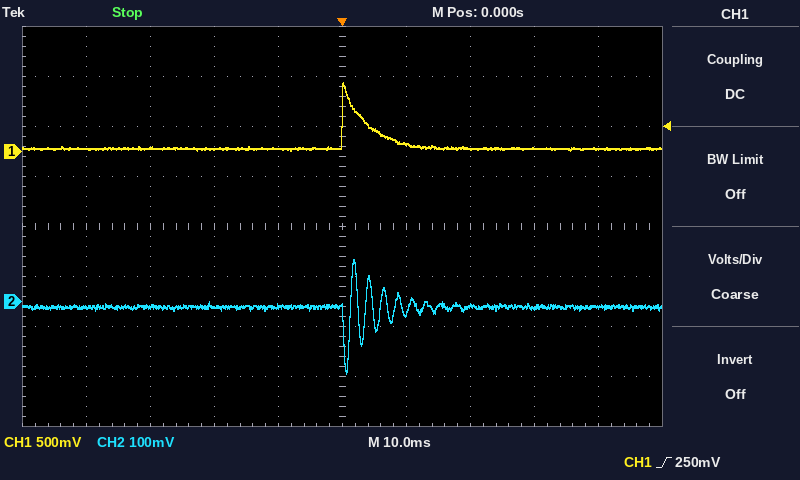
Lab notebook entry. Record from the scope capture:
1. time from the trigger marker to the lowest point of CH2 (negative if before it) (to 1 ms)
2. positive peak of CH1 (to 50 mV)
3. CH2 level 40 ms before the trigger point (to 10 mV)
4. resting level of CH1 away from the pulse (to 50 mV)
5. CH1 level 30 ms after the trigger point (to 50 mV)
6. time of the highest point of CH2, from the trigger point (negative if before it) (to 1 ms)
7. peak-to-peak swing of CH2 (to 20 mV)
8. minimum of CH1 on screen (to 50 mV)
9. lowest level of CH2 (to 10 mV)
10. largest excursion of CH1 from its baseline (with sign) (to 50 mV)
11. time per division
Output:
+1 ms
700 mV
-10 mV
50 mV
50 mV
+2 ms
220 mV
0 mV
-140 mV
+650 mV
10 ms
